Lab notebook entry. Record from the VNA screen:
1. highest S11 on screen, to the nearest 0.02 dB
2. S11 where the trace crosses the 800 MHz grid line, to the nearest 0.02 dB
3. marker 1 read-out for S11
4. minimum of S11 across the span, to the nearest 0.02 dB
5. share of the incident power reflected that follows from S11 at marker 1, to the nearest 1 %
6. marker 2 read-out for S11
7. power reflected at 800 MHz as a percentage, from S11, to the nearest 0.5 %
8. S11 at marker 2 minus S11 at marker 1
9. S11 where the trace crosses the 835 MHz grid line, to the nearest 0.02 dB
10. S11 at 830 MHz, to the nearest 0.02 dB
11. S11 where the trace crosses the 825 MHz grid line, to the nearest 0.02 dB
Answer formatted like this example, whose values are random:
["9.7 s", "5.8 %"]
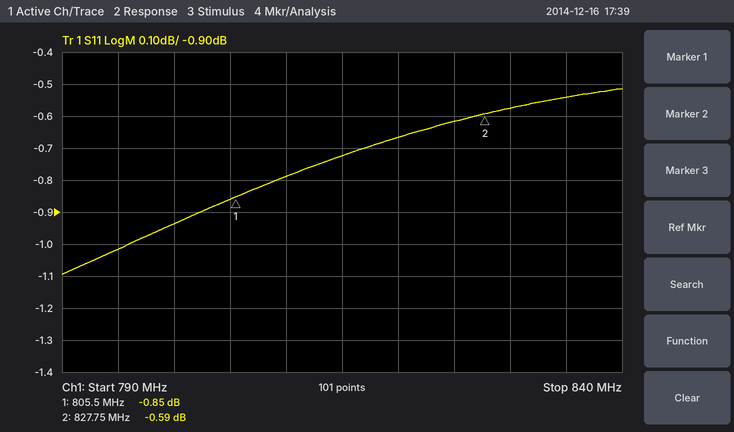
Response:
["-0.52 dB", "-0.94 dB", "-0.85 dB", "-1.10 dB", "82 %", "-0.59 dB", "80.5 %", "0.26 dB", "-0.54 dB", "-0.58 dB", "-0.62 dB"]
